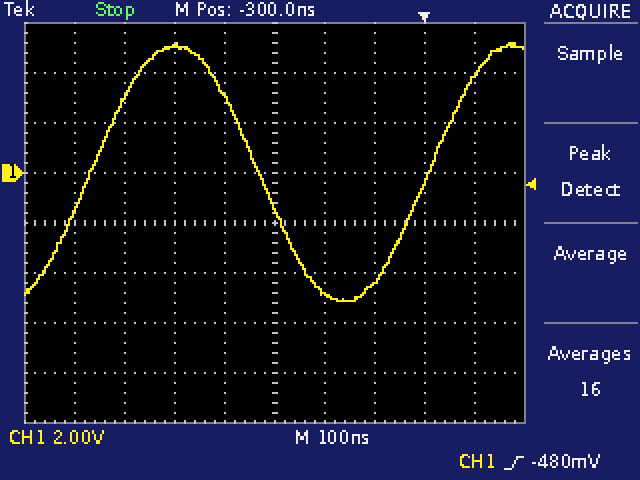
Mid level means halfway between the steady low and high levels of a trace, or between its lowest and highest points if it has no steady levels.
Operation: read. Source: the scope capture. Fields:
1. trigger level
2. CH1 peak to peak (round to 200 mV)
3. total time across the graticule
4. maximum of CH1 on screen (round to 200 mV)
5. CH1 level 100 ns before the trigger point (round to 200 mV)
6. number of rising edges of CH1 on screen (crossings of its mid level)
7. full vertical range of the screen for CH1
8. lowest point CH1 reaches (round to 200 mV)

-480 mV
10.4 V
1 µs
5.2 V
-4.4 V
2
16 V
-5.2 V
